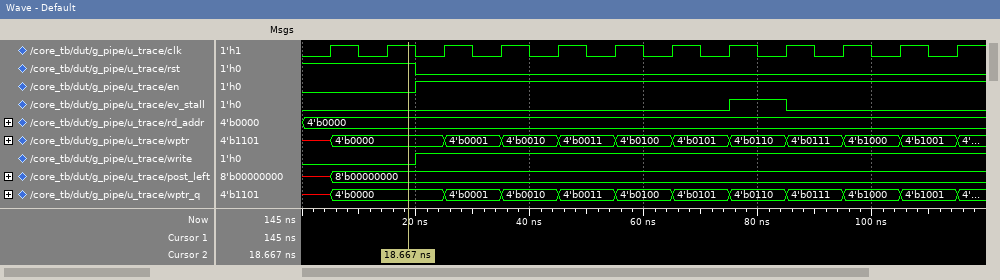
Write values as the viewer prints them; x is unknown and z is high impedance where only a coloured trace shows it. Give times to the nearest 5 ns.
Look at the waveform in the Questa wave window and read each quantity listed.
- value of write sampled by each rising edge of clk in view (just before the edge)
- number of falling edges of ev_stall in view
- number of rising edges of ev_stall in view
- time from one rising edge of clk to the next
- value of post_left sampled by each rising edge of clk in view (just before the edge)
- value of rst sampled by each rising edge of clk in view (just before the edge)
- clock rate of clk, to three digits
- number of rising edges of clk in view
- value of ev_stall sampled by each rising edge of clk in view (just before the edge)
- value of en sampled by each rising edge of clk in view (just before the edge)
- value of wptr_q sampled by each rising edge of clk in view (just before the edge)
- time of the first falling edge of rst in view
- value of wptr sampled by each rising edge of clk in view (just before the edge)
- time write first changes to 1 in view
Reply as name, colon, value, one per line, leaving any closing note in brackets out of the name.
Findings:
value of write sampled by each rising edge of clk in view: 0 0 1 1 1 1 1 1 1 1 1 1
number of falling edges of ev_stall in view: 1
number of rising edges of ev_stall in view: 1
time from one rising edge of clk to the next: 10 ns
value of post_left sampled by each rising edge of clk in view: x, 8'b00000000, 8'b00000000, 8'b00000000, 8'b00000000, 8'b00000000, 8'b00000000, 8'b00000000, 8'b00000000, 8'b00000000, 8'b00000000, 8'b00000000
value of rst sampled by each rising edge of clk in view: 1 1 0 0 0 0 0 0 0 0 0 0
clock rate of clk, to three digits: 100 MHz
number of rising edges of clk in view: 12
value of ev_stall sampled by each rising edge of clk in view: 0 0 0 0 0 0 0 0 1 0 0 0
value of en sampled by each rising edge of clk in view: 0 0 1 1 1 1 1 1 1 1 1 1
value of wptr_q sampled by each rising edge of clk in view: x, 4'b0000, 4'b0000, 4'b0001, 4'b0010, 4'b0011, 4'b0100, 4'b0101, 4'b0110, 4'b0111, 4'b1000, 4'b1001
time of the first falling edge of rst in view: 20 ns
value of wptr sampled by each rising edge of clk in view: x, 4'b0000, 4'b0000, 4'b0001, 4'b0010, 4'b0011, 4'b0100, 4'b0101, 4'b0110, 4'b0111, 4'b1000, 4'b1001
time write first changes to 1 in view: 20 ns
